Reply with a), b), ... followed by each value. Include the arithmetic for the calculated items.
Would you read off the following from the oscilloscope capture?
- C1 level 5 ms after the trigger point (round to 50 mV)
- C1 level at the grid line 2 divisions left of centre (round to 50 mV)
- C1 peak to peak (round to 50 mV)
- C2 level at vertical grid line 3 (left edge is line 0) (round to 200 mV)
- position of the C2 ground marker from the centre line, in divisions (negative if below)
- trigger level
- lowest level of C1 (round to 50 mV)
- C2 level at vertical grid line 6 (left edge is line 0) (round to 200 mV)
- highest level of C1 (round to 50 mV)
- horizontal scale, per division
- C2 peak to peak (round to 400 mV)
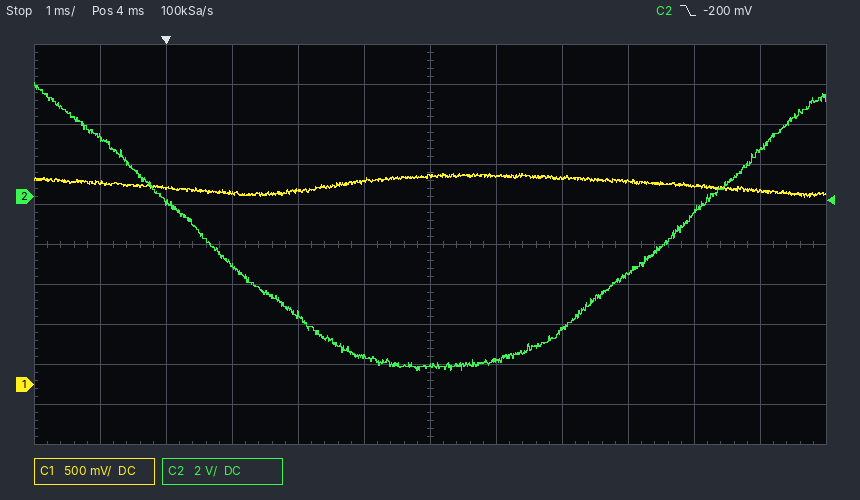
a) 2.60 V
b) 2.40 V
c) 2.65 V − (2.35 V) = 300 mV
d) -3.4 V
e) +1.2 div
f) -200 mV
g) 2.35 V
h) -8.4 V
i) 2.65 V
j) 1 ms
k) 14.4 V
